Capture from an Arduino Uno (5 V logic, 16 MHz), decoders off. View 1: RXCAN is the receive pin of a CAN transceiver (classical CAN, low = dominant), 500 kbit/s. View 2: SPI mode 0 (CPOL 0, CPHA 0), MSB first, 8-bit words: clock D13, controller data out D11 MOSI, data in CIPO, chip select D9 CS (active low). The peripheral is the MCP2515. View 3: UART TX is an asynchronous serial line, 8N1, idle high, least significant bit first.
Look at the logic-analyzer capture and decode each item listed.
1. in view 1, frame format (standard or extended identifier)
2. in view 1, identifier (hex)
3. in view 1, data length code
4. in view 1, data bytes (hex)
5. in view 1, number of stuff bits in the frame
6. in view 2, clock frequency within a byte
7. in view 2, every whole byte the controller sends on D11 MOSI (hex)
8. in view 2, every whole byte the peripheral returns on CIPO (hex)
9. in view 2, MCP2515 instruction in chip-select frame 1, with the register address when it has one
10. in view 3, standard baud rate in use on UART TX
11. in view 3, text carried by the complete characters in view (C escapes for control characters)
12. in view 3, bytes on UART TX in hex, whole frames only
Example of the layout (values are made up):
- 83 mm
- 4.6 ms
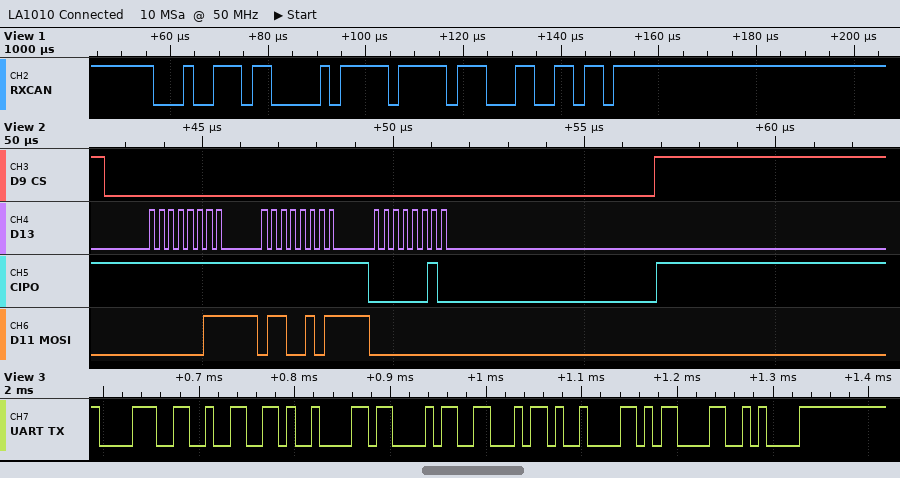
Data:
- standard
- 0x13B
- 1
- FF
- 3
- 4 MHz
- 03 65 00
- FF FF 02
- READ 0x65
- 115200 baud
- "82\tCF\t\r\n"
- 38 32 09 43 46 09 0D 0A
